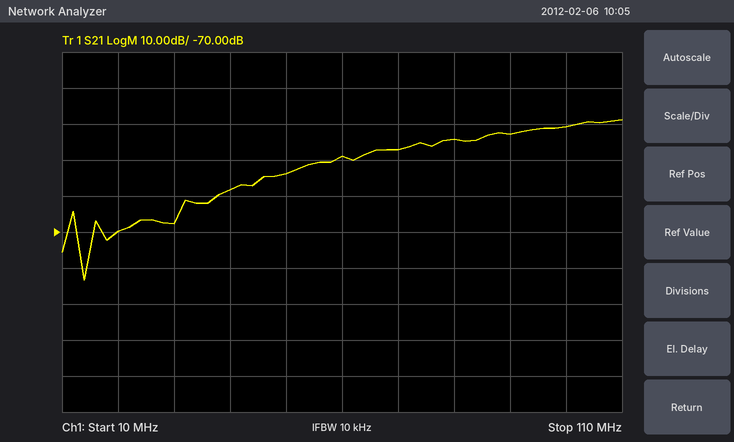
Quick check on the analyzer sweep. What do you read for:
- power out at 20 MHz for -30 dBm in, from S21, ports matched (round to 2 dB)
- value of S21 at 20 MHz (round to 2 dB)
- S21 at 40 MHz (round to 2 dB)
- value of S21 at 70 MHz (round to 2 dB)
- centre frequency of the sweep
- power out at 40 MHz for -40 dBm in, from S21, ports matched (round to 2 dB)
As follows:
-100 dBm
-70 dB
-58 dB
-48 dB
60 MHz
-98 dBm
